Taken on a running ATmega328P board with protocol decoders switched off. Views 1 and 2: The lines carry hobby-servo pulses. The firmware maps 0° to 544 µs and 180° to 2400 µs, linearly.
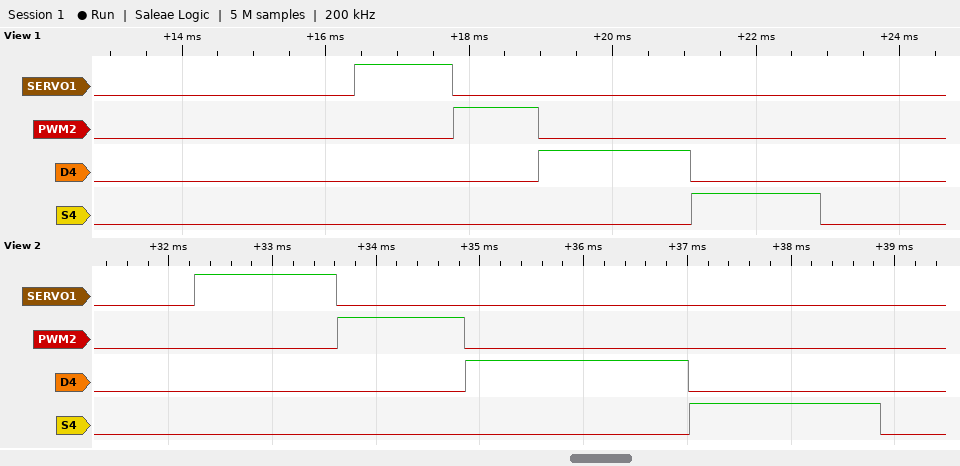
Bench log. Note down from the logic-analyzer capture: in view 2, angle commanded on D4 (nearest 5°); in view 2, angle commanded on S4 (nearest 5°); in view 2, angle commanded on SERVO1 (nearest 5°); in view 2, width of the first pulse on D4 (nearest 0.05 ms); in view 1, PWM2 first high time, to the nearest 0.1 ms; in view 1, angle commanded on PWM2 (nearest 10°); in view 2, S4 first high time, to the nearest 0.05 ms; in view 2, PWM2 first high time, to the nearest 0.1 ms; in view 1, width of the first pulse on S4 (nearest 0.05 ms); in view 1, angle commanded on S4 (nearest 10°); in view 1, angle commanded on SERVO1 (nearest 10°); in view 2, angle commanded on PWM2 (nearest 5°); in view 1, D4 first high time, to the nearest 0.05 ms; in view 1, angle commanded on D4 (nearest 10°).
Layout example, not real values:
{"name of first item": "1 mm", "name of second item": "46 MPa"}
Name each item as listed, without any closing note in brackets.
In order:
{"in view 2, angle commanded on D4": "155°", "in view 2, angle commanded on S4": "125°", "in view 2, angle commanded on SERVO1": "80°", "in view 2, width of the first pulse on D4": "2.15 ms", "in view 1, PWM2 first high time, to the nearest 0.1 ms": "1.2 ms", "in view 1, angle commanded on PWM2": "60°", "in view 2, S4 first high time, to the nearest 0.05 ms": "1.85 ms", "in view 2, PWM2 first high time, to the nearest 0.1 ms": "1.2 ms", "in view 1, width of the first pulse on S4": "1.80 ms", "in view 1, angle commanded on S4": "120°", "in view 1, angle commanded on SERVO1": "80°", "in view 2, angle commanded on PWM2": "65°", "in view 1, D4 first high time, to the nearest 0.05 ms": "2.10 ms", "in view 1, angle commanded on D4": "150°"}
